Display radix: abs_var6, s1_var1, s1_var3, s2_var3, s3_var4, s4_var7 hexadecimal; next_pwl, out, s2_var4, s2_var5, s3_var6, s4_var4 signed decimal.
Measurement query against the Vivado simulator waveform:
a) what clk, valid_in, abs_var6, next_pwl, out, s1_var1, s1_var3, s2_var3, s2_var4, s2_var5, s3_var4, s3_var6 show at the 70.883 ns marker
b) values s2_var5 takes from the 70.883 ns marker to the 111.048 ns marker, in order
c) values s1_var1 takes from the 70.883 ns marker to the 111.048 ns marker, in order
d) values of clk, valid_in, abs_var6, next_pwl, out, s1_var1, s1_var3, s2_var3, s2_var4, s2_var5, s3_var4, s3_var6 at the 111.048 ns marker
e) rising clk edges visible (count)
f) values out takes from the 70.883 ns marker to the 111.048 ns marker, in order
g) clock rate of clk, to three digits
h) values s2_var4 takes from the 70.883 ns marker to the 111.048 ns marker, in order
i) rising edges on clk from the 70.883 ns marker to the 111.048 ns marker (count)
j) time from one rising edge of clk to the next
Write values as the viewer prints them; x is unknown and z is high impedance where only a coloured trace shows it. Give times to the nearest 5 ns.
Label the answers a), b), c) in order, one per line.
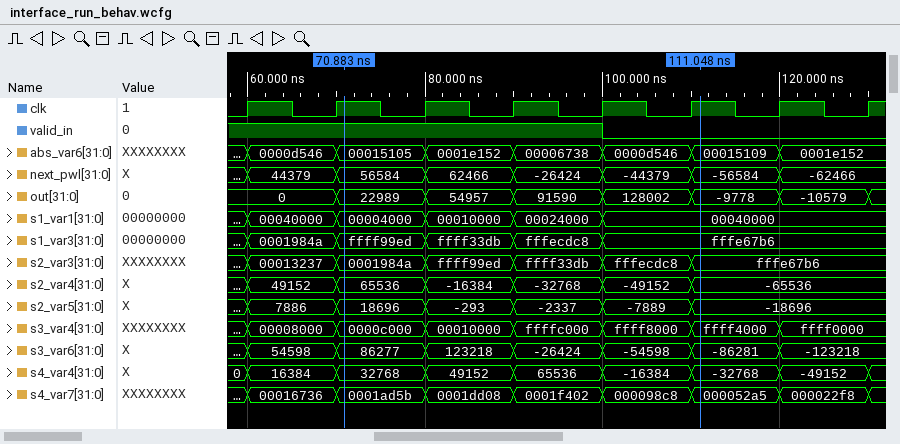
a) clk=1, valid_in=1, abs_var6=00015105, next_pwl=56584, out=22989, s1_var1=00004000, s1_var3=ffff99ed, s2_var3=0001984a, s2_var4=65536, s2_var5=18696, s3_var4=0000c000, s3_var6=86277
b) 18696, -293, -2337, -7889, -18696
c) 00004000, 00010000, 00024000, 00040000
d) clk=1, valid_in=0, abs_var6=00015109, next_pwl=-56584, out=-9778, s1_var1=00040000, s1_var3=fffe67b6, s2_var3=fffe67b6, s2_var4=-65536, s2_var5=-18696, s3_var4=ffff4000, s3_var6=-86281
e) 8
f) 22989, 54957, 91590, 128002, -9778
g) 100 MHz
h) 65536, -16384, -32768, -49152, -65536
i) 4
j) 10 ns
